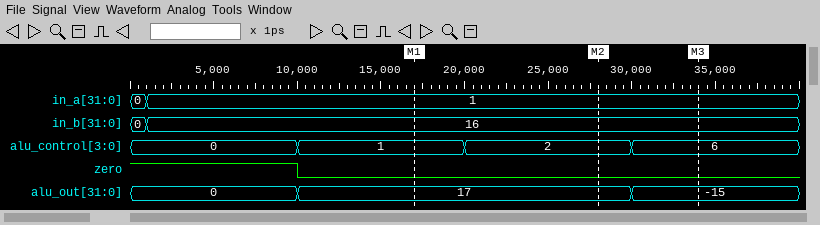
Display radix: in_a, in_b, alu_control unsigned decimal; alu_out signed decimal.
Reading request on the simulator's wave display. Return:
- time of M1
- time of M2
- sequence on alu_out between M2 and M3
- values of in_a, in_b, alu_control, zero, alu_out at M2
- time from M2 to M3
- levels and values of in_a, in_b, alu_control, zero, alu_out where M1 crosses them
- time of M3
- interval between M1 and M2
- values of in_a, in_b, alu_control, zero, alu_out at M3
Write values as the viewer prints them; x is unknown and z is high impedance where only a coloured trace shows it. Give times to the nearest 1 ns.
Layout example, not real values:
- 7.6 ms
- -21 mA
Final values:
- 17 ns
- 28 ns
- 17, -15
- in_a=1, in_b=16, alu_control=2, zero=0, alu_out=17
- 6 ns
- in_a=1, in_b=16, alu_control=1, zero=0, alu_out=17
- 34 ns
- 11 ns
- in_a=1, in_b=16, alu_control=6, zero=0, alu_out=-15
